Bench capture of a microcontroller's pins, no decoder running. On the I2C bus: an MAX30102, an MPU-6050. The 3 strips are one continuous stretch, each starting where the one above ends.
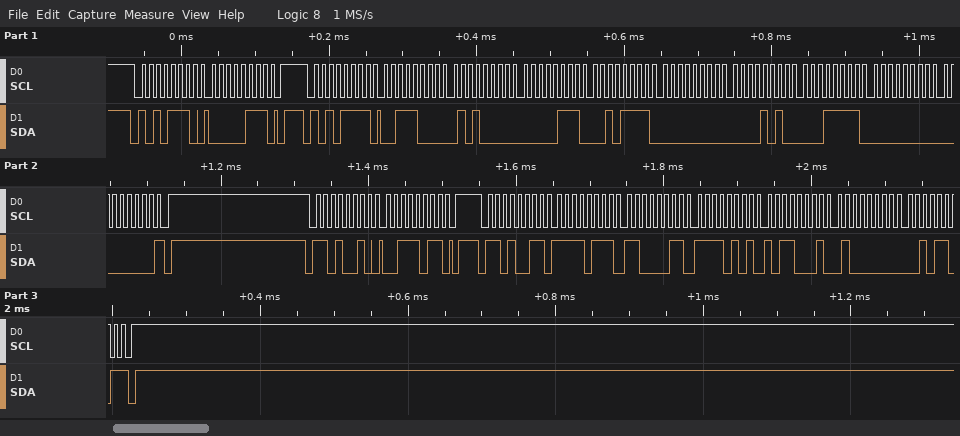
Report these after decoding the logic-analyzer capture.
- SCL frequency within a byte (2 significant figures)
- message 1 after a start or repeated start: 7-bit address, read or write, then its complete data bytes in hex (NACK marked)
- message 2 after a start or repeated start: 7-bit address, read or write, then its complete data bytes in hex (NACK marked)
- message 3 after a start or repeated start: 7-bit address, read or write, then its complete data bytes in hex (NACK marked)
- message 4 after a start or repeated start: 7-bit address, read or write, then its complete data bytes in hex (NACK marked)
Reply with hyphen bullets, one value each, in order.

- 100 kHz
- 0x57 write: 07
- 0x57 read: 38 50 07 2F 00 0A 1F 00 00 NACK
- 0x69 write: 3B
- 0x69 read: F7 C3 F5 B1 40 2D NACK
